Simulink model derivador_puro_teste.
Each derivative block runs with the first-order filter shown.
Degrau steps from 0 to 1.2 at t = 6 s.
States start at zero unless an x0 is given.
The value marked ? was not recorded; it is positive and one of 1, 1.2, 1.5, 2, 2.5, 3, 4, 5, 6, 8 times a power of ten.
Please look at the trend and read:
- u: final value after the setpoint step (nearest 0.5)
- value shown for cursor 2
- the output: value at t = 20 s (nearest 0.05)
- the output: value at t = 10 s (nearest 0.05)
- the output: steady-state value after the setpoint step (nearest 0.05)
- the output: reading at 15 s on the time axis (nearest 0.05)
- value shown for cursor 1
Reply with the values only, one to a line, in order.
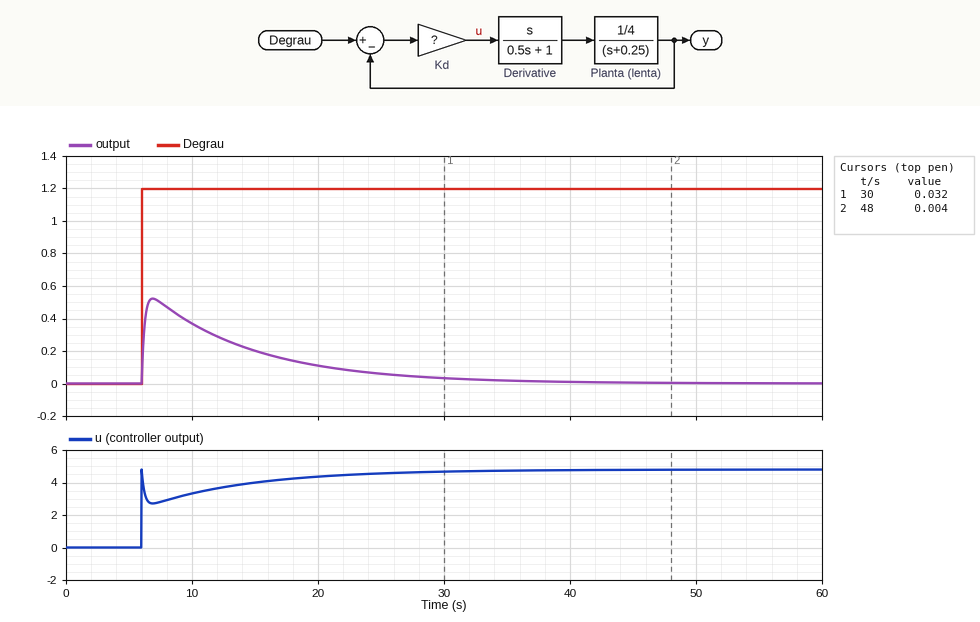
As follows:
5.0
0.004
0.10
0.35
0.00
0.20
0.032
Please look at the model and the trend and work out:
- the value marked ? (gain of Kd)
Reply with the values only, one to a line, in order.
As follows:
4
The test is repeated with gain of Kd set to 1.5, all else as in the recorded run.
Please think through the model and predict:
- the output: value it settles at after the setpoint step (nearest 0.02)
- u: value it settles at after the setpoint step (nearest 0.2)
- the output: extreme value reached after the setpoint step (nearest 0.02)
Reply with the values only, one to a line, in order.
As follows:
0.00
1.8
0.26
